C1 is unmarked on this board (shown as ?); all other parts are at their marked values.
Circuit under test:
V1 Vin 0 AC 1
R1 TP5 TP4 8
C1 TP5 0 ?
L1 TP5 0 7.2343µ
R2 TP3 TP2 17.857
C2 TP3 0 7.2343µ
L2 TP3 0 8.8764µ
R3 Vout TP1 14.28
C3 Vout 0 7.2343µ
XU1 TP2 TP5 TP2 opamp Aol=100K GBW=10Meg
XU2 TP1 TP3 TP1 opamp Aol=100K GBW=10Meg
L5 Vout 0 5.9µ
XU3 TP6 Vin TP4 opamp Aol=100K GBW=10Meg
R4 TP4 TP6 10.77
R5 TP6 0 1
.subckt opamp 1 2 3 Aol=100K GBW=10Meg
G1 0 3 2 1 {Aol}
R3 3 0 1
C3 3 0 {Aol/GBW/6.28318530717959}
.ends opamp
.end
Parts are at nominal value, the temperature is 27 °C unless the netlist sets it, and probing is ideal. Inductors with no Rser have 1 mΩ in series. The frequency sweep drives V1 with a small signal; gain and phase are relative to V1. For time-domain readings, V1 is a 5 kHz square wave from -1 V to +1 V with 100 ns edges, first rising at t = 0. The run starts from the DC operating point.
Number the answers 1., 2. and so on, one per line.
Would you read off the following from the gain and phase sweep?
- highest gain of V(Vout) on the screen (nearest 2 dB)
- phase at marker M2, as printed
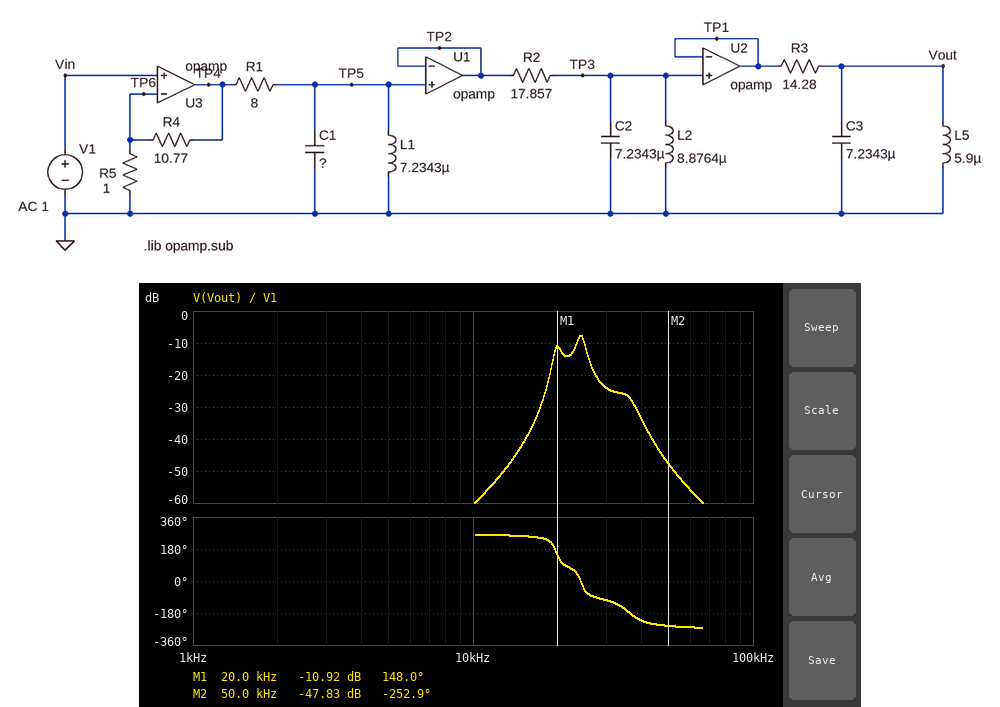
1. -8 dB
2. -252.9 deg
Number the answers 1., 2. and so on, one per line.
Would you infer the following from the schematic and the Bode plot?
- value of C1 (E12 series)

1. 2.7 µF
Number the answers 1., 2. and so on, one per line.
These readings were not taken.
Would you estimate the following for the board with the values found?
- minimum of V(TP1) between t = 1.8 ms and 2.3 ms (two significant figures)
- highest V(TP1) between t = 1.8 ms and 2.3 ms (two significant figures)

1. -260 mV
2. 260 mV
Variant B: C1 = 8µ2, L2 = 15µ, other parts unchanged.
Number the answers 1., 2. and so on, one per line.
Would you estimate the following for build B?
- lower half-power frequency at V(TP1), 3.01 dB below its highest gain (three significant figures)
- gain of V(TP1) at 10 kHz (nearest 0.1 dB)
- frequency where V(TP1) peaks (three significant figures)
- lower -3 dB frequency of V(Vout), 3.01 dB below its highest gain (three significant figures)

1. 14.8 kHz
2. -21.9 dB
3. 15.4 kHz
4. 20.0 kHz
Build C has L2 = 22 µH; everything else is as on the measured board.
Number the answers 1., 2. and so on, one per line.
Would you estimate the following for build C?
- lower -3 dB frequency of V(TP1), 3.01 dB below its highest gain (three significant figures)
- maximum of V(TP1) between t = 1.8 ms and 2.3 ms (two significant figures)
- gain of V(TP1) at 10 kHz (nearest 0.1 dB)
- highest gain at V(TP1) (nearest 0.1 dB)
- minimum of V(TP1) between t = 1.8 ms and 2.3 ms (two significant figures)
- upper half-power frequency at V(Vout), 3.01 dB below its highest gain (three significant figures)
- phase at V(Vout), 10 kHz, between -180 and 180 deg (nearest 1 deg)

1. 12.1 kHz
2. 290 mV
3. -16.6 dB
4. -0.4 dB
5. -290 mV
6. 25.2 kHz
7. -108 deg
